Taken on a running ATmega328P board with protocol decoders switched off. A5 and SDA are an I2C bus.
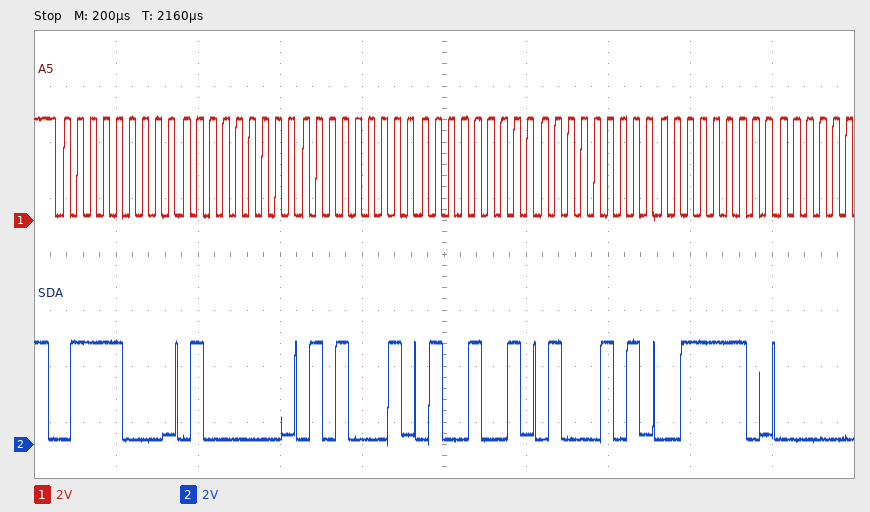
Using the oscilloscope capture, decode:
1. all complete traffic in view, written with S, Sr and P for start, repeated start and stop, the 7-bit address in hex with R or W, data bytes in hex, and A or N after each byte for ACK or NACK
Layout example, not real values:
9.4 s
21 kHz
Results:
S 3CW A 40 A 51 A 49 A 45 A 3E A
